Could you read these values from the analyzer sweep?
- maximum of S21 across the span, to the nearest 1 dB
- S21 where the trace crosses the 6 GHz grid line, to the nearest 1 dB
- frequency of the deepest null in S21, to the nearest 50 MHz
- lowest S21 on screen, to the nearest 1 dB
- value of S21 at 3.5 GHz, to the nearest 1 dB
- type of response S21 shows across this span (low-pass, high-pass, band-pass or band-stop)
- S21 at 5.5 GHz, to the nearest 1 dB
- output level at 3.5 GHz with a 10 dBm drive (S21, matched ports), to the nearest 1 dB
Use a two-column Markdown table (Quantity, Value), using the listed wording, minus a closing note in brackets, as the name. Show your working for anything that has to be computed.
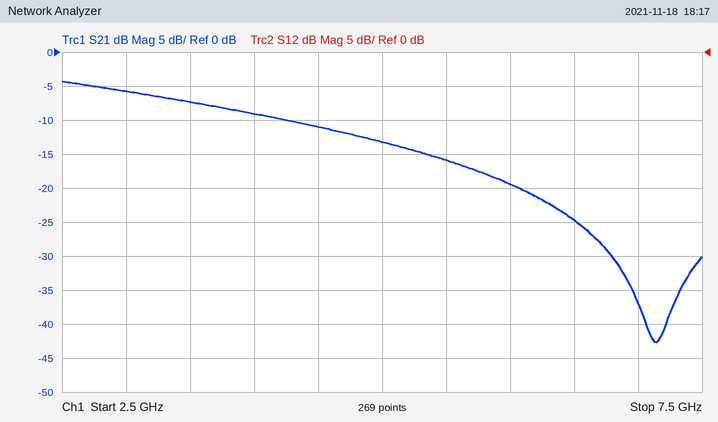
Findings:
| Quantity | Value |
|---|---|
| maximum of S21 across the span, to the nearest 1 dB | -4 dB |
| S21 where the trace crosses the 6 GHz grid line, to the nearest 1 dB | -19 dB |
| frequency of the deepest null in S21, to the nearest 50 MHz | 7.15 GHz |
| lowest S21 on screen, to the nearest 1 dB | -43 dB |
| value of S21 at 3.5 GHz, to the nearest 1 dB | -7 dB |
| type of response S21 shows across this span | low-pass |
| S21 at 5.5 GHz, to the nearest 1 dB | -16 dB |
| output level at 3.5 GHz with a 10 dBm drive (S21, matched ports), to the nearest 1 dB | 10 dBm + (-7 dB) = 3 dBm |
